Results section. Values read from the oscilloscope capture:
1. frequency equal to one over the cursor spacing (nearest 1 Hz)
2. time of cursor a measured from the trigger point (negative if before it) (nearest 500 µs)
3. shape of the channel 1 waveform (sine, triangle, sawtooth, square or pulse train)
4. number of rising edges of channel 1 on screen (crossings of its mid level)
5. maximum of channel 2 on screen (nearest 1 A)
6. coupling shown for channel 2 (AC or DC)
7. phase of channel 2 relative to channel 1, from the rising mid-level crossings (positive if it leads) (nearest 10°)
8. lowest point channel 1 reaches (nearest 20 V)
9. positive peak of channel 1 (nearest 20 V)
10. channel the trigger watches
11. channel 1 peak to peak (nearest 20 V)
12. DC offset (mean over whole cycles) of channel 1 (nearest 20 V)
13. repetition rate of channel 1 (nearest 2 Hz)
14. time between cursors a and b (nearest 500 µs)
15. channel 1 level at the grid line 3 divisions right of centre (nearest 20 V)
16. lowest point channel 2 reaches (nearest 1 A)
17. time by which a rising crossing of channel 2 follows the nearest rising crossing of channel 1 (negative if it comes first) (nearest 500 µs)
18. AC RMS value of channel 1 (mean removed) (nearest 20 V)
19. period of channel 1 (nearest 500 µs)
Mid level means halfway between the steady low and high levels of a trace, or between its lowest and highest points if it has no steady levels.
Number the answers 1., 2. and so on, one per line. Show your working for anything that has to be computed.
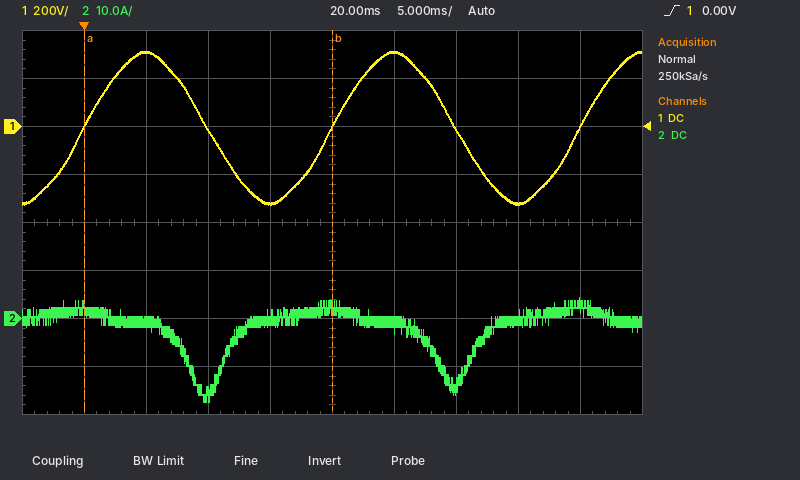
1. 1 / 20.0 ms ≈ 50 Hz
2. 0.0 ms
3. sine
4. 3
5. 4 A
6. DC
7. −360° × (-8.5 ms) / 20.0 ms ≈ +153°, so +150° to the nearest 10°
8. -320 V
9. 320 V
10. channel 1
11. 320 V − (-320 V) = 640 V
12. (320 V + (-320 V)) / 2 ≈ 0 V
13. 1 / 20.0 ms ≈ 50 Hz
14. 20.0 ms
15. -320 V
16. -17 A
17. -8.5 ms
18. 640 V / (2√2) ≈ 226 V, so 220 V to the nearest 20 V
19. 20.0 ms
